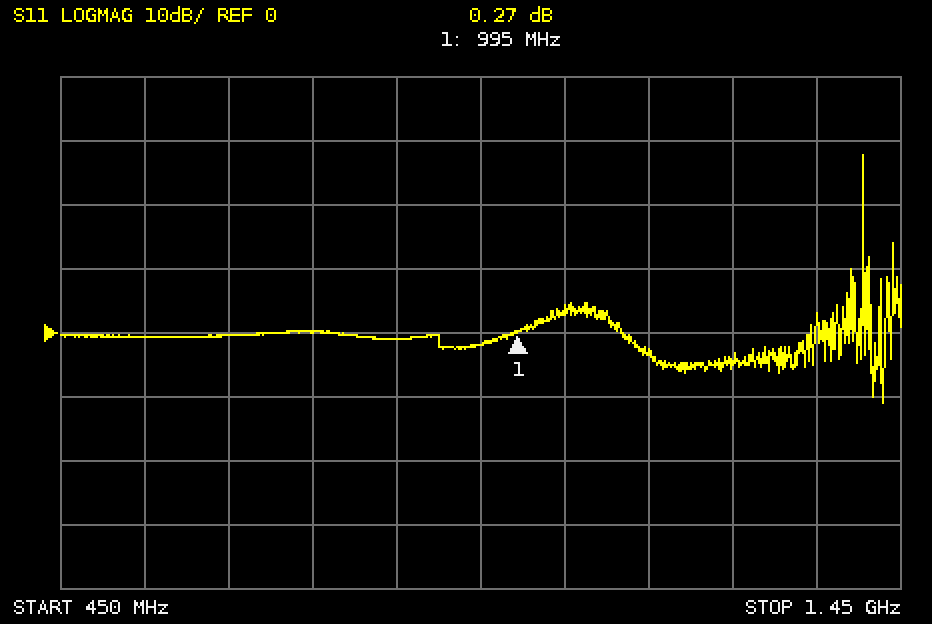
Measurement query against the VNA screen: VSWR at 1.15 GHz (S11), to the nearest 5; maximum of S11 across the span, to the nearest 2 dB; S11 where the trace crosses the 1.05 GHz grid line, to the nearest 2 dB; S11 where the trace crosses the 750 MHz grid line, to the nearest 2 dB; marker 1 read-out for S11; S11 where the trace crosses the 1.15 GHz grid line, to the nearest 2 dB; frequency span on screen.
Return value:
5
28 dB
4 dB
0 dB
0.27 dB
-4 dB
1 GHz
